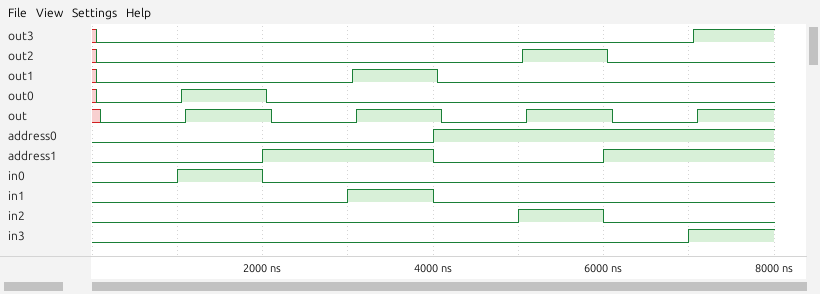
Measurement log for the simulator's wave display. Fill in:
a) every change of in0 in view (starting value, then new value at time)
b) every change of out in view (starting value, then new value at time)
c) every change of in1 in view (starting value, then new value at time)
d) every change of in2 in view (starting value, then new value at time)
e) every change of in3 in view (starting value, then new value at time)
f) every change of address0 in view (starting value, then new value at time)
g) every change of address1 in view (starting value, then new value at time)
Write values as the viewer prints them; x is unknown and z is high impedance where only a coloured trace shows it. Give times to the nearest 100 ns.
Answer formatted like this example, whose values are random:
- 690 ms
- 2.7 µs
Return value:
- 0, 1 at 1000 ns, 0 at 2000 ns
- x, 0 at 100 ns, 1 at 1100 ns, 0 at 2100 ns, 1 at 3100 ns, 0 at 4100 ns, 1 at 5100 ns, 0 at 6100 ns, 1 at 7100 ns
- 0, 1 at 3000 ns, 0 at 4000 ns
- 0, 1 at 5000 ns, 0 at 6000 ns
- 0, 1 at 7000 ns
- 0, 1 at 4000 ns
- 0, 1 at 2000 ns, 0 at 4000 ns, 1 at 6000 ns
